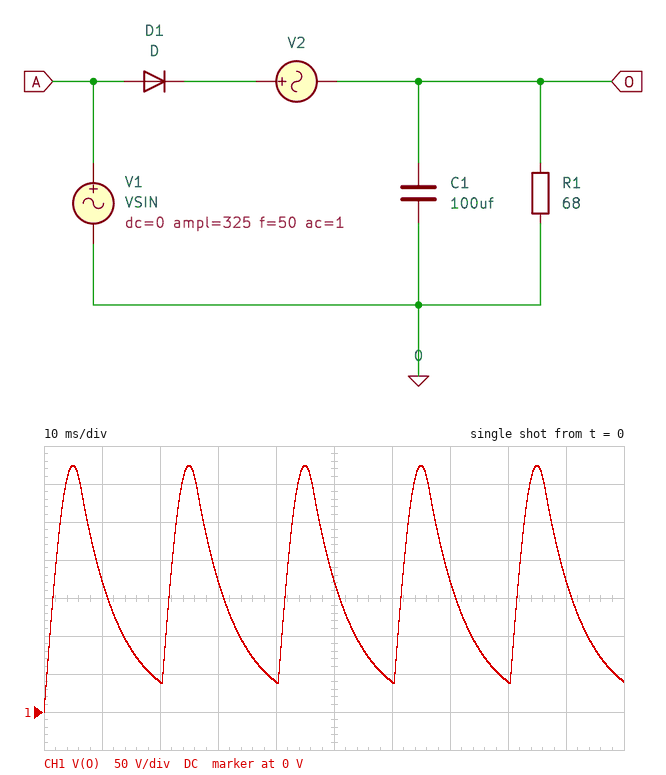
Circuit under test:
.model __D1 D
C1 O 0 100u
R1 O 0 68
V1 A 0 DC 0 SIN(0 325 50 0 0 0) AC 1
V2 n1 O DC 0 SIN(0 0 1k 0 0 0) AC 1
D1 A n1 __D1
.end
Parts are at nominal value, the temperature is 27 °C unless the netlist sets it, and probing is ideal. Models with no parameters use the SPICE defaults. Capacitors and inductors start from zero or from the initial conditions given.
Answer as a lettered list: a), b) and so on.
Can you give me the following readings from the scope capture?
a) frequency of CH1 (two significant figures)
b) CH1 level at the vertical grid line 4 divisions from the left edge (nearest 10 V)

a) 50 Hz
b) 40 V
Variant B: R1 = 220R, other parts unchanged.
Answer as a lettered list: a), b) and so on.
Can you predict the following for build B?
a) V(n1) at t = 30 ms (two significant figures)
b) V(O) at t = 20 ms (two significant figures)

a) 260 V
b) 170 V
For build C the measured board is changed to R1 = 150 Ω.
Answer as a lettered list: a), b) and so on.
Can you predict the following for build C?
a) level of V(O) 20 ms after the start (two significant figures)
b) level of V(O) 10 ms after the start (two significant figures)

a) 120 V
b) 240 V
